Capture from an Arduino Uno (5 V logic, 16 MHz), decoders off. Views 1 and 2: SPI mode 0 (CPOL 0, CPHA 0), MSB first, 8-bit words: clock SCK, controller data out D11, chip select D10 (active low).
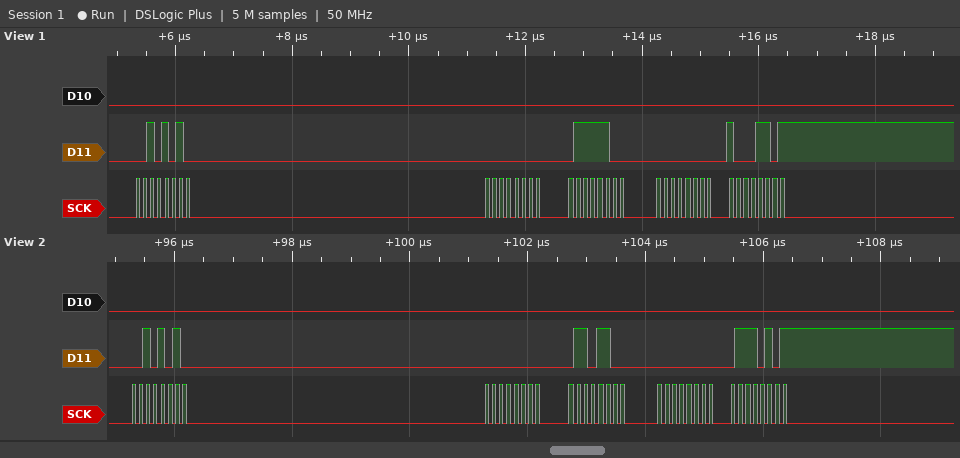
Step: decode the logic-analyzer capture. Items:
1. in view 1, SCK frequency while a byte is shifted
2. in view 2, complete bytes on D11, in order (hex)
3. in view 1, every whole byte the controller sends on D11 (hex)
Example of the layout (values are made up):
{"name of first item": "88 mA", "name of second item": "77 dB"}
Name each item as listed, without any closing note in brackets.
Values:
{"in view 1, SCK frequency while a byte is shifted": "8 MHz", "in view 2, complete bytes on D11, in order": "2A 00 6C 00 75", "in view 1, every whole byte the controller sends on D11": "2A 00 7C 00 8D"}
